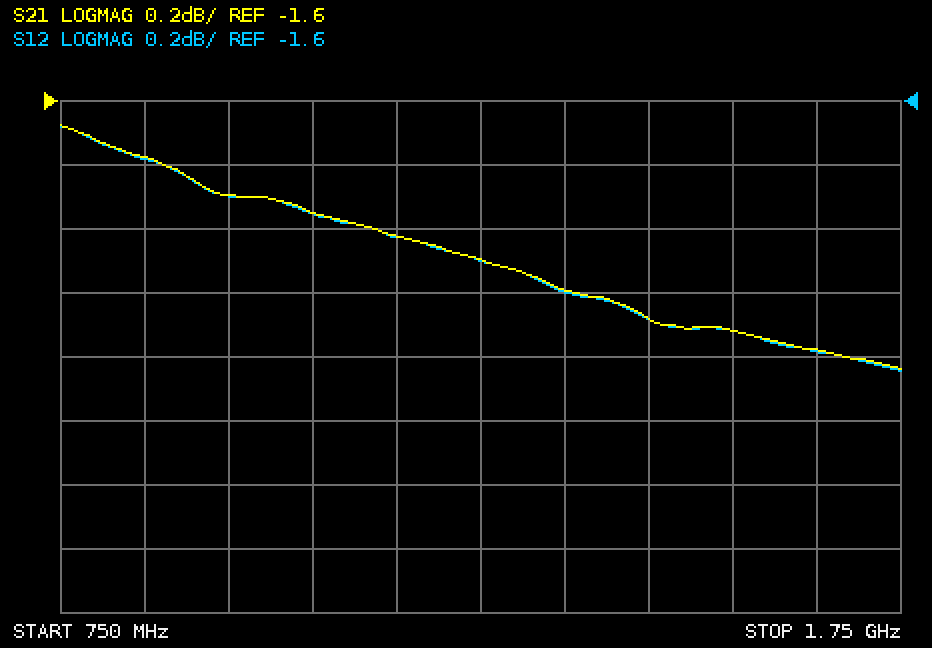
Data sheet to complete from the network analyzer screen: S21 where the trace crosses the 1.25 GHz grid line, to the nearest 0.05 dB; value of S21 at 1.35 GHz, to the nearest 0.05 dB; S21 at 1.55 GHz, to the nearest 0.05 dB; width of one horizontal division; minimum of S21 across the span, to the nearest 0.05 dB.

-2.10 dB
-2.20 dB
-2.30 dB
100 MHz
-2.45 dB
